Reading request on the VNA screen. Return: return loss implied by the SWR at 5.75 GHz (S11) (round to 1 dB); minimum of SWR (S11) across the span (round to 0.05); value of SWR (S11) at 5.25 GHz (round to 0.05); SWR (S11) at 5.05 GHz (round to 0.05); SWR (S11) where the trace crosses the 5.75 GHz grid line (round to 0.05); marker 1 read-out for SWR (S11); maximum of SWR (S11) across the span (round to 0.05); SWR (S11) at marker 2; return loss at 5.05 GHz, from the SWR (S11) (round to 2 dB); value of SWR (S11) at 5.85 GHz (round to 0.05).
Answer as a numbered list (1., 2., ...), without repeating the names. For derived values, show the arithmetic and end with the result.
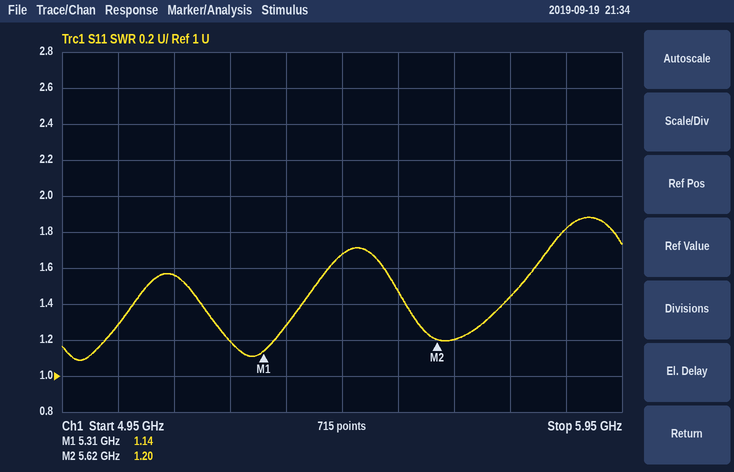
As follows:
1. −20 log10((1.45 − 1)/(1.45 + 1)) ≈ 15 dB
2. 1.10
3. 1.20
4. 1.30
5. 1.45
6. 1.14
7. 1.90
8. 1.20
9. −20 log10((1.3 − 1)/(1.3 + 1)) ≈ 18 dB
10. 1.80
